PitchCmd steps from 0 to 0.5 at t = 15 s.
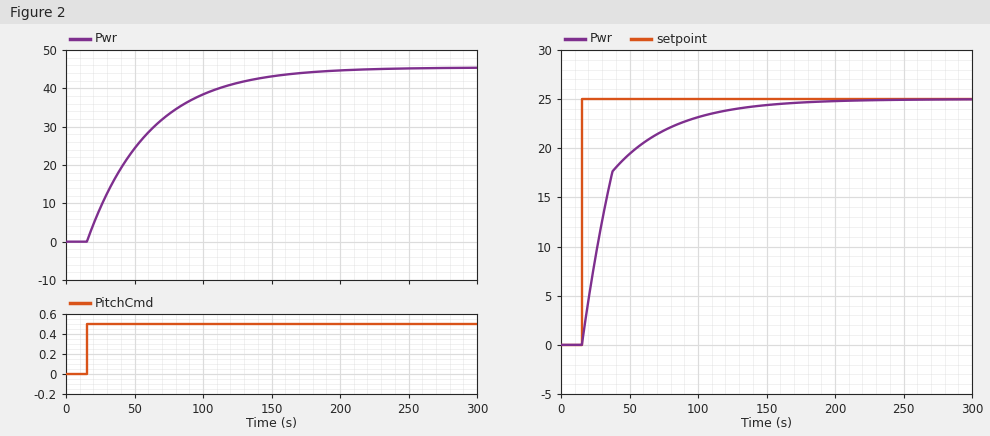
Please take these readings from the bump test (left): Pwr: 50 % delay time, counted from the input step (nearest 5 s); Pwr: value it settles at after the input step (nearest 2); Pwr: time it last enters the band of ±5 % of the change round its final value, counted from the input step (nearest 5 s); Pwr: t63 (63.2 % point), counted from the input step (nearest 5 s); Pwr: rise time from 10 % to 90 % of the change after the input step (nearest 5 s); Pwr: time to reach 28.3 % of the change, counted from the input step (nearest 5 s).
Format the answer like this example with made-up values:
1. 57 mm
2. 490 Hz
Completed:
1. 30 s
2. 46
3. 135 s
4. 45 s
5. 100 s
6. 15 s
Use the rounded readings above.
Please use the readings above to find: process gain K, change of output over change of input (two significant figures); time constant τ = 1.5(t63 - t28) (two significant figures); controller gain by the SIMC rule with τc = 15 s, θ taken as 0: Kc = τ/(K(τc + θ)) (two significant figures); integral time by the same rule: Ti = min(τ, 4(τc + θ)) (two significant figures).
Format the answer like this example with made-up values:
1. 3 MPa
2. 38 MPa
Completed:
1. 92
2. 45 s
3. 0.033
4. 45 s
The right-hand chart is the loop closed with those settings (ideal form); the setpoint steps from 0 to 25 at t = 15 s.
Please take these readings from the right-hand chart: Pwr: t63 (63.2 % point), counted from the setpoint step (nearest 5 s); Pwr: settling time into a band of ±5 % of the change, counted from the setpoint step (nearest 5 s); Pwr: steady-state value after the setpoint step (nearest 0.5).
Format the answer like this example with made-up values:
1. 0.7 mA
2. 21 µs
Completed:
1. 20 s
2. 100 s
3. 25.0
